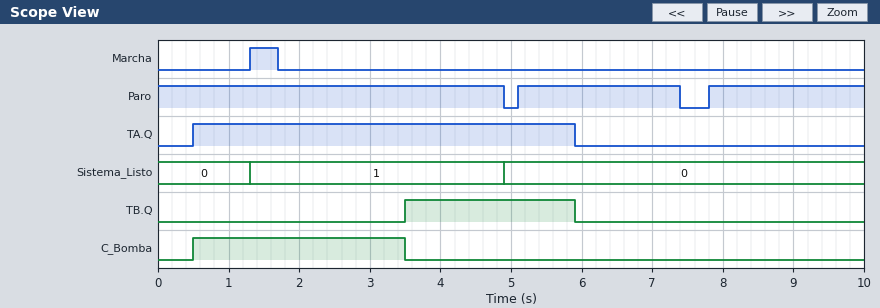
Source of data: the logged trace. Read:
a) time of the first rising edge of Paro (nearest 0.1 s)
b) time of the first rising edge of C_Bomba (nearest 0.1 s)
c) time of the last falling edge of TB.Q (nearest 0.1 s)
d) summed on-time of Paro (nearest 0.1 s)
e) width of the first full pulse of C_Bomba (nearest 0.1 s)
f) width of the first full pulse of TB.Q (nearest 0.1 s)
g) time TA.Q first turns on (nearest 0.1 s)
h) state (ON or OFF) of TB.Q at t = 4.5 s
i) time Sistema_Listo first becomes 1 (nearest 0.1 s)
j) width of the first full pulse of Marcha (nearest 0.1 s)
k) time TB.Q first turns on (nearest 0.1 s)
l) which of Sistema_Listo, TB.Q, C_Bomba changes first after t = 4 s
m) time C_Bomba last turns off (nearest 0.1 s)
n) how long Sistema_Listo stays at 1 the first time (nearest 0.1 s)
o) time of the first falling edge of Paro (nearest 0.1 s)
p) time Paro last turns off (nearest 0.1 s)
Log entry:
5.1 s
0.5 s
5.9 s
9.4 s
3.0 s
2.4 s
0.5 s
ON
1.3 s
0.4 s
3.5 s
Sistema_Listo
3.5 s
3.6 s
4.9 s
7.4 s
